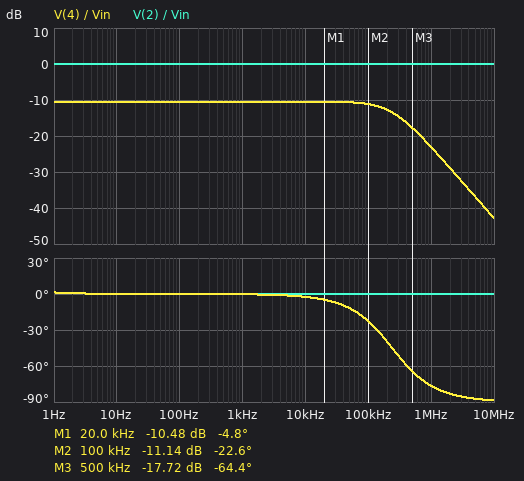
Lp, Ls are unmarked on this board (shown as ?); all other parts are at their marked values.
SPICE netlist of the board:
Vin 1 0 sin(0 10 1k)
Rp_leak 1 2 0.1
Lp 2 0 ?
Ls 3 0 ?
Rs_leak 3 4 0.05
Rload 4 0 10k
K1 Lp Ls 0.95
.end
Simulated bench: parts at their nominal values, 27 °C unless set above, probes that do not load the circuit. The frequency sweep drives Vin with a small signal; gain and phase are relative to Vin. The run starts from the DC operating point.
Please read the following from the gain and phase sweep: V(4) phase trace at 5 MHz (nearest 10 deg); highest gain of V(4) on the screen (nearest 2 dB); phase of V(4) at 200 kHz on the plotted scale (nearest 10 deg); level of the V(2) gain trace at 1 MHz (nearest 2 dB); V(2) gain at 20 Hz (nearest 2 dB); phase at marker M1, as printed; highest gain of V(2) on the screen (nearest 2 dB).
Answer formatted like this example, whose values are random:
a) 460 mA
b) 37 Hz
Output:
a) -90 deg
b) -10 dB
c) -40 deg
d) 0 dB
e) 0 dB
f) -4.8 deg
g) 0 dB
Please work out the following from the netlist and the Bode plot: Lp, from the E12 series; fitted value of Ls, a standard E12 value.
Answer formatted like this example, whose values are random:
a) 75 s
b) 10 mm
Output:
a) 680 mH
b) 68 mH
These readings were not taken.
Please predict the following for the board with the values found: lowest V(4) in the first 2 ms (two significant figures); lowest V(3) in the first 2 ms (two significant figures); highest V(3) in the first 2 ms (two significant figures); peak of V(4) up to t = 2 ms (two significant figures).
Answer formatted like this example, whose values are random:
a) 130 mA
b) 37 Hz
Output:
a) -3.0 V
b) -3.0 V
c) 3.0 V
d) 3.0 V
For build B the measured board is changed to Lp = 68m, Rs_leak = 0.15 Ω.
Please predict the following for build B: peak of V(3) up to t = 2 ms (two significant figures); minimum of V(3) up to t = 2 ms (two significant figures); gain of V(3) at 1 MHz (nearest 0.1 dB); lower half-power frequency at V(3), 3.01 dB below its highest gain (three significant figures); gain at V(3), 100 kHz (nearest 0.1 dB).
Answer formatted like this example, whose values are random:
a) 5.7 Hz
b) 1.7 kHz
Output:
a) 9.5 V
b) -9.5 V
c) -13.1 dB
d) 234 mHz
e) -1.1 dB
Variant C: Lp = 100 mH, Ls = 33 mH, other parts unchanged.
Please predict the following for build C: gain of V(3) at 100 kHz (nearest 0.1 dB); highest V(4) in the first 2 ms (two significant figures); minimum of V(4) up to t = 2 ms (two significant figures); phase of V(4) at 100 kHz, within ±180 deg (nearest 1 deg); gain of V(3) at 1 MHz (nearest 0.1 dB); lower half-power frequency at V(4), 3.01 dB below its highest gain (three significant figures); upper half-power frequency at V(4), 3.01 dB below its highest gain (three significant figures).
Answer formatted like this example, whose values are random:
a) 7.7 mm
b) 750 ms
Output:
a) -5.4 dB
b) 5.5 V
c) -5.5 V
d) -11 deg
e) -12.3 dB
f) 159 mHz
g) 495 kHz
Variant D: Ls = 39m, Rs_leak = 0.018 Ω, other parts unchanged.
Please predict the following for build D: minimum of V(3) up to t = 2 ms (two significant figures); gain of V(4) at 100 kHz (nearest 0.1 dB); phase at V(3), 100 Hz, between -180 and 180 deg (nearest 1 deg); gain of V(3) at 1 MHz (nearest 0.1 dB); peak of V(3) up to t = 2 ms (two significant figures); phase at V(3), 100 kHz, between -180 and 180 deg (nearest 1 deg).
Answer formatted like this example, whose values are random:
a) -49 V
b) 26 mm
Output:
a) -2.3 V
b) -13.1 dB
c) 0 deg
d) -21.1 dB
e) 2.3 V
f) -13 deg
